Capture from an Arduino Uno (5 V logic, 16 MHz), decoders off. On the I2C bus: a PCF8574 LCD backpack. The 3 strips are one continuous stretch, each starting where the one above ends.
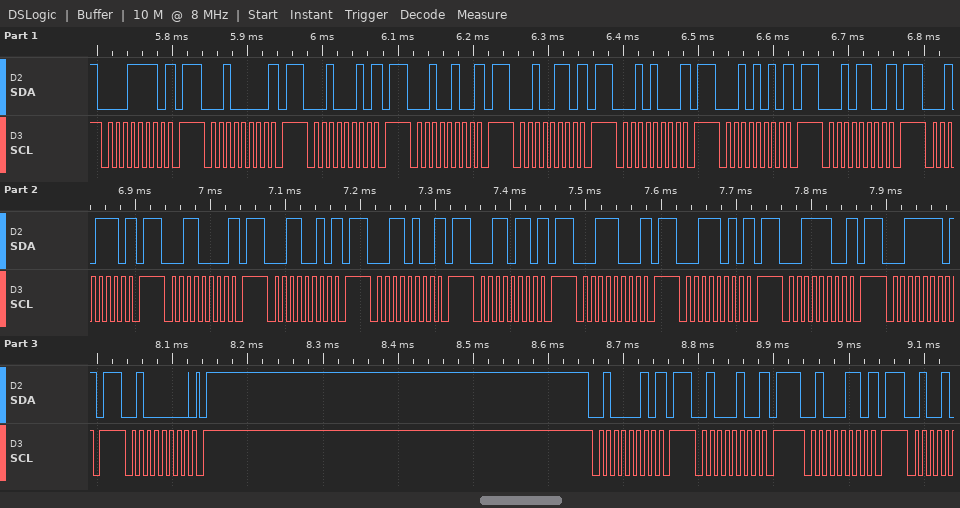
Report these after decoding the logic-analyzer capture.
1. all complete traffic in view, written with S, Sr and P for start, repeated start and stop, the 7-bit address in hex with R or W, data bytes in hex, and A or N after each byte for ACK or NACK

S 0FW N P S 10W N P S 11W N P S 12W N P S 13W N P S 14W N P S 15W N P S 16W N P S 17W N P S 18W N P S 19W N P S 1AW N P S 1BW N P S 1CW N P S 1DW N P S 1EW N P S 1FW N P S 20W A P S 21W N P S 22W N P S 23W N P
